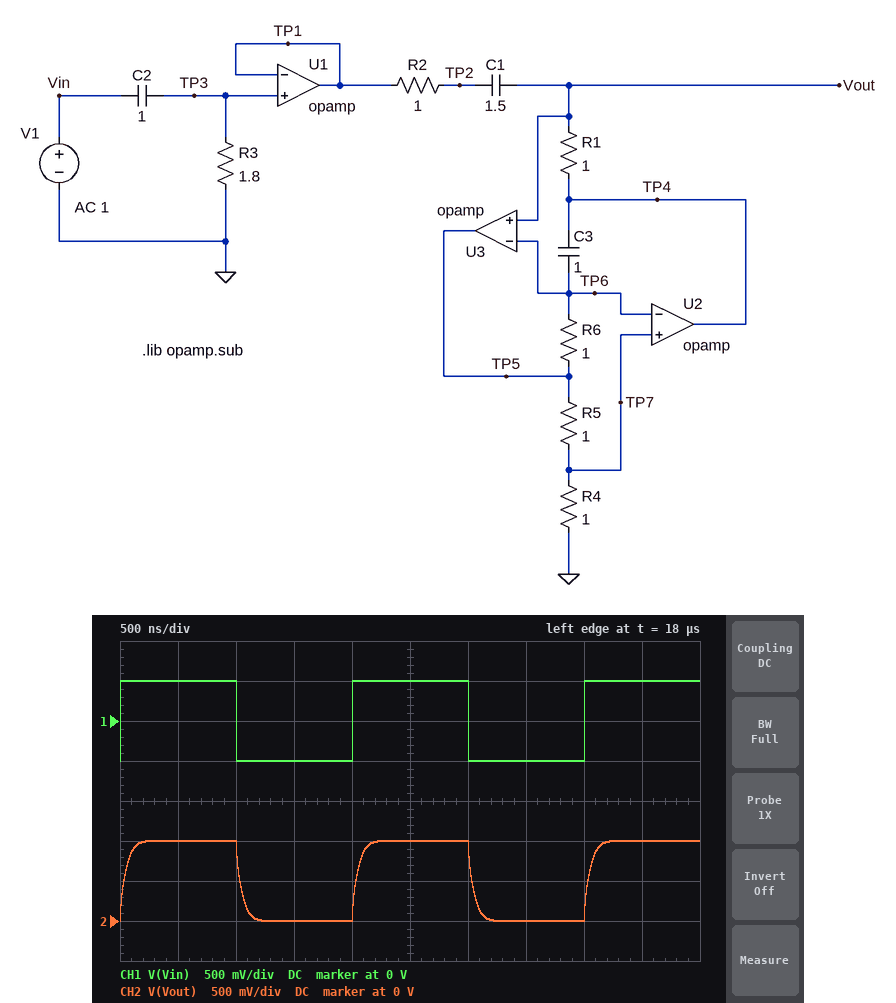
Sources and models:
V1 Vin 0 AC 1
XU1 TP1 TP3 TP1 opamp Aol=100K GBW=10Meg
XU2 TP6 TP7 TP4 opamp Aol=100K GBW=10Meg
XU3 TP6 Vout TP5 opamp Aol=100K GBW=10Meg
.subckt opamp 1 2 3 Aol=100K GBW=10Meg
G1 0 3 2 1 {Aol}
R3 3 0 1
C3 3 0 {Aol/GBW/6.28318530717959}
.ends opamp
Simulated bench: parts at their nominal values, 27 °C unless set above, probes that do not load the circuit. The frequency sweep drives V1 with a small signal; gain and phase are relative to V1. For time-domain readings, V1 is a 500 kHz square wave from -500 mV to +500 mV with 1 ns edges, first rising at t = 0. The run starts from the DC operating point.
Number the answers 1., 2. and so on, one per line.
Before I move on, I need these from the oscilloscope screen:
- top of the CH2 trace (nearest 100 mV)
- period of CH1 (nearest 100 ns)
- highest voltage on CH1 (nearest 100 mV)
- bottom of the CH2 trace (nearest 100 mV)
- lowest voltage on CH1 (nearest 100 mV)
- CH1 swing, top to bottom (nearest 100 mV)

1. 1.0 V
2. 2.0 µs
3. 500 mV
4. 0 V
5. -500 mV
6. 1.0 V
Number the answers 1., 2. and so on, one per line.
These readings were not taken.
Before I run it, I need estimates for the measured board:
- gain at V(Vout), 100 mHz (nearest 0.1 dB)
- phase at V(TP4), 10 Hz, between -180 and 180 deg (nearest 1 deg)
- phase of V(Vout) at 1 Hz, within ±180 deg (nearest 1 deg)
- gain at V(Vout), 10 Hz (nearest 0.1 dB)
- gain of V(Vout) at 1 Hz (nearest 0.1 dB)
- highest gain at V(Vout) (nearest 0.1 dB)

1. -7.3 dB
2. 2 deg
3. 14 deg
4. 0 dB
5. 0 dB
6. 0 dB
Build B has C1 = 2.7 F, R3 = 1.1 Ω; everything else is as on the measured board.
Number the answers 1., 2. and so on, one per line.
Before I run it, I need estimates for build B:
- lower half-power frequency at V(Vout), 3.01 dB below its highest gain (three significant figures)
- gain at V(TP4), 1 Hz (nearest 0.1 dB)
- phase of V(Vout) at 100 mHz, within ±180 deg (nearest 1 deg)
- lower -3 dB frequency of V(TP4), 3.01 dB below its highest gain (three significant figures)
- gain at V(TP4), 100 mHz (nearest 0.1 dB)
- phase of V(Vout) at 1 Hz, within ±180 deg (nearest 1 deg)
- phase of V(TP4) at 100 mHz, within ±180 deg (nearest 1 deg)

1. 188 mHz
2. 0 dB
3. 143 deg
4. 106 mHz
5. -3.5 dB
6. 17 deg
7. -159 deg
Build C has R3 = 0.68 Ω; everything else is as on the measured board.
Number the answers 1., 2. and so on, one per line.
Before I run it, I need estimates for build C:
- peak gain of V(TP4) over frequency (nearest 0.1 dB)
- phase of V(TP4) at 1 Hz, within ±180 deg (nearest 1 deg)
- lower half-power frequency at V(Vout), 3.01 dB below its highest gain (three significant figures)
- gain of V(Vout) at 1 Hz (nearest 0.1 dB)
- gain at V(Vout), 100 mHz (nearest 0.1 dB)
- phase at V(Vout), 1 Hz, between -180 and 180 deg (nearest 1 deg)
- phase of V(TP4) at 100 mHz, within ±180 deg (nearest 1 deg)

1. 0 dB
2. 31 deg
3. 222 mHz
4. -0.2 dB
5. -12.9 dB
6. 22 deg
7. -122 deg
